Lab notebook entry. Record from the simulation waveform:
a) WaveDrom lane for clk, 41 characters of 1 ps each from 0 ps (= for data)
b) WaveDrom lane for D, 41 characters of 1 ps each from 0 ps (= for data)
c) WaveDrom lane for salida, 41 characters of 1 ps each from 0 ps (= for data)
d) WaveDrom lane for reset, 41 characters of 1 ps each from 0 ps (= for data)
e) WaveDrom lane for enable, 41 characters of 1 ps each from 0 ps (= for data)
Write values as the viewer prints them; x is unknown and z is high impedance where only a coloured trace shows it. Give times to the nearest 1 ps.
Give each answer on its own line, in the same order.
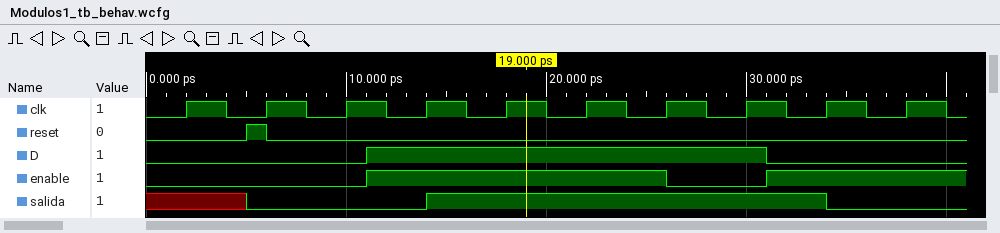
{name: 'clk', wave: '0.1.0.1.0.1.0.1.0.1.0.1.0.1.0.1.0.1.0.1.0'}
{name: 'D', wave: '0..........1...................0.........'}
{name: 'salida', wave: 'x....0........1...................0......'}
{name: 'reset', wave: '0....10..................................'}
{name: 'enable', wave: '0..........1..............0....1.........'}
